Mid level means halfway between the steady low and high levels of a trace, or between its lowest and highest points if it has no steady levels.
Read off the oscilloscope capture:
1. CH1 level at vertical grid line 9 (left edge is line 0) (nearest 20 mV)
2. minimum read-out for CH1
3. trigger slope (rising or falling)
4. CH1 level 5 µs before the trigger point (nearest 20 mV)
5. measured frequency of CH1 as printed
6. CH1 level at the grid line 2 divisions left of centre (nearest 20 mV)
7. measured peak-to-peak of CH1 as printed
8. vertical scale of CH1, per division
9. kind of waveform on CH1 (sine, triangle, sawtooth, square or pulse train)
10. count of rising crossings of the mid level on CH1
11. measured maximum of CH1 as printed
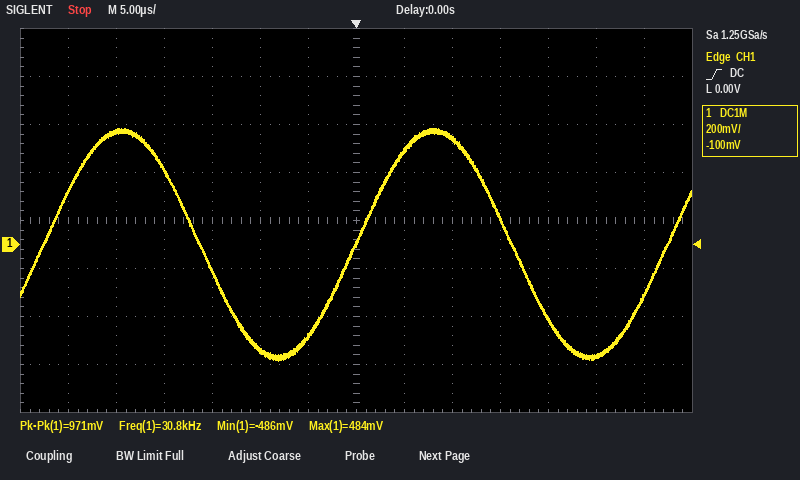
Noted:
440 mV
-486 mV
rising
-380 mV
30.8 kHz
-440 mV
971 mV
200 mV
sine
3
484 mV
